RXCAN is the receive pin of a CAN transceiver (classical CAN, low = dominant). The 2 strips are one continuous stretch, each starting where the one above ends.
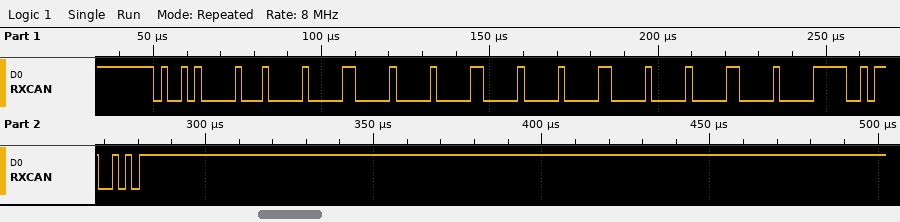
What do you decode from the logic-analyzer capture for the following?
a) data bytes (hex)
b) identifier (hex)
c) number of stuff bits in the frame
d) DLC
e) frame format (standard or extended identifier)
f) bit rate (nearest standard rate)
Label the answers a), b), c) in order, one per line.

a) 01 00 01 00 01 00 01 00
b) 0x4A0
c) 15
d) 8
e) standard
f) 500 kbit/s
